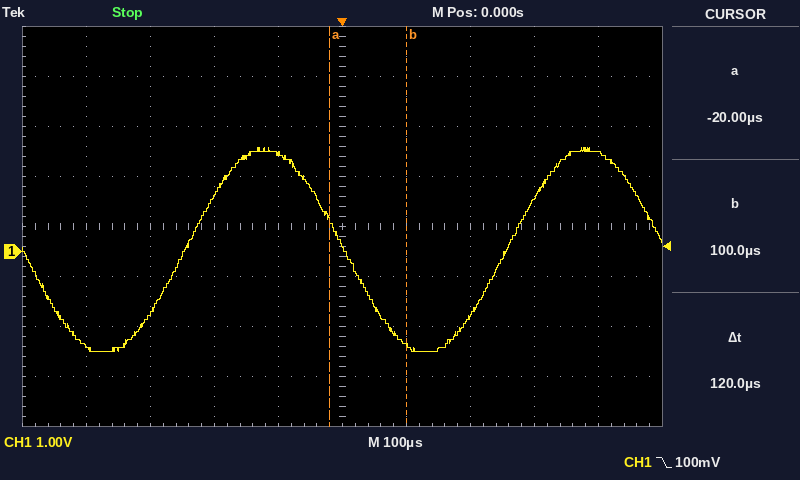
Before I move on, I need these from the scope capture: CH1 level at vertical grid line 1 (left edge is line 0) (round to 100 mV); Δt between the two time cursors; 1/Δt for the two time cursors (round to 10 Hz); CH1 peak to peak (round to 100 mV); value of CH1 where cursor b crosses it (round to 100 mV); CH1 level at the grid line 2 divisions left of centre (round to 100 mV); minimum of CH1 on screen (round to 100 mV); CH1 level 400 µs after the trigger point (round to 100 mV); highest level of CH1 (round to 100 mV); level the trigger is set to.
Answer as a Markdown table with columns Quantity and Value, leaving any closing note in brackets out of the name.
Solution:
| Quantity | Value |
|---|---|
| CH1 level at vertical grid line 1 (left edge is line 0) | -1.9 V |
| Δt between the two time cursors | 120 µs |
| 1/Δt for the two time cursors | 8.33 kHz |
| CH1 peak to peak | 4.1 V |
| value of CH1 where cursor b crosses it | -1.9 V |
| CH1 level at the grid line 2 divisions left of centre | 1.1 V |
| minimum of CH1 on screen | -2.0 V |
| CH1 level 400 µs after the trigger point | 2.0 V |
| highest level of CH1 | 2.1 V |
| level the trigger is set to | 100 mV |
